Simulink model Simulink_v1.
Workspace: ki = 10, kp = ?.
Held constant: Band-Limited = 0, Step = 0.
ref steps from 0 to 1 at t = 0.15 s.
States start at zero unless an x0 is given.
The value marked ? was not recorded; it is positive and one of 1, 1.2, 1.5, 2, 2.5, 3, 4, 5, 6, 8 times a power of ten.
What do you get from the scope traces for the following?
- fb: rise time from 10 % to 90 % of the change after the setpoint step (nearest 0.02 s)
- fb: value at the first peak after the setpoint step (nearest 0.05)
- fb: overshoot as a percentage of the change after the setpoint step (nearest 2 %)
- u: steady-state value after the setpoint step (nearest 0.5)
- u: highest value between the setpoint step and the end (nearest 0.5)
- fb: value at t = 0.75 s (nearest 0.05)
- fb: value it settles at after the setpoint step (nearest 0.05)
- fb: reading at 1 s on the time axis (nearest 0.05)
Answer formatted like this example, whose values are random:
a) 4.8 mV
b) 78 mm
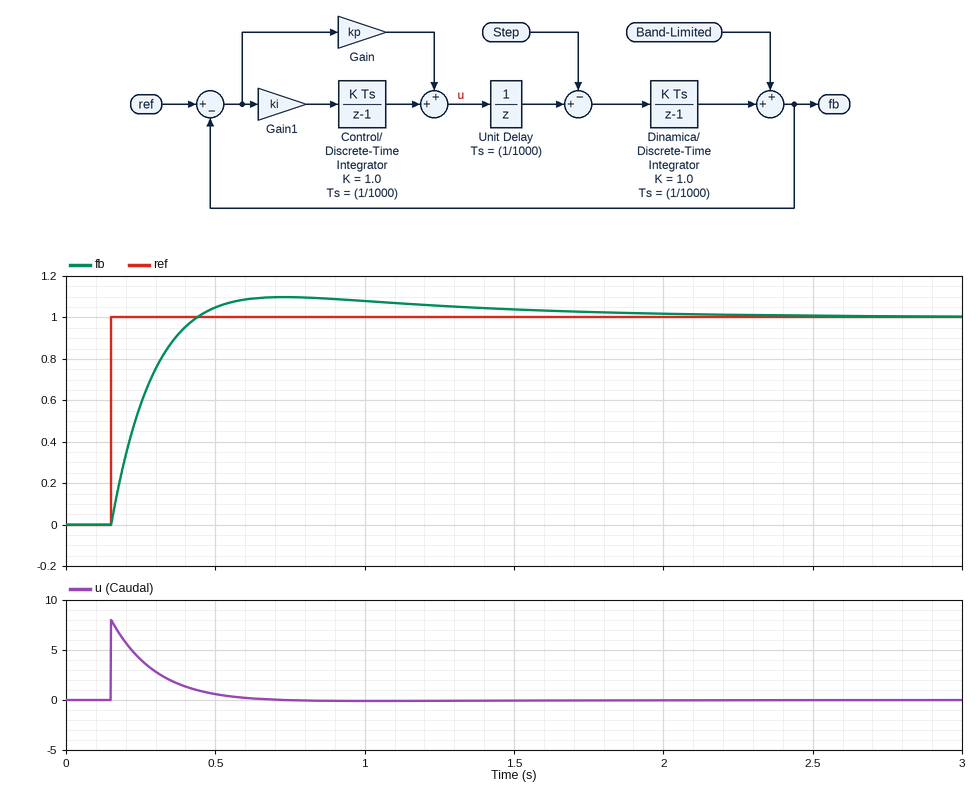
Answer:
a) 0.20 s
b) 1.10
c) 10 %
d) 0.0
e) 8.0
f) 1.10
g) 1.00
h) 1.10
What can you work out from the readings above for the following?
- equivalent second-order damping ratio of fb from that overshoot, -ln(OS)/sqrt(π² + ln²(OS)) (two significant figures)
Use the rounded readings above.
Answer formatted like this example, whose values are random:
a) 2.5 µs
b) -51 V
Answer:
a) 0.59
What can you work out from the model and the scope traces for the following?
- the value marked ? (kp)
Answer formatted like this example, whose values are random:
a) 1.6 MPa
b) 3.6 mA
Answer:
a) 8
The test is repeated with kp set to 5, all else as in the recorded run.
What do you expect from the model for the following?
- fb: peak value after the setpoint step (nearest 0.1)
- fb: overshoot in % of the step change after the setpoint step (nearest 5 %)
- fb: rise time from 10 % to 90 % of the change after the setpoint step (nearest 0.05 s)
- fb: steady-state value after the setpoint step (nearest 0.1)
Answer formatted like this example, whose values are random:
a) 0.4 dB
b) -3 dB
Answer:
a) 1.2
b) 20 %
c) 0.25 s
d) 1.0
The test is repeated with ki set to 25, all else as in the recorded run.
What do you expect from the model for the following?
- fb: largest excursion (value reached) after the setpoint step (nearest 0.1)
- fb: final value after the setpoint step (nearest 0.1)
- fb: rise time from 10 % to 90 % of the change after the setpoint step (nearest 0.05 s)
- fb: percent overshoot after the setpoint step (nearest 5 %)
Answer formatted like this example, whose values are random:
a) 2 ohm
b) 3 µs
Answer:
a) 1.2
b) 1.0
c) 0.15 s
d) 20 %
